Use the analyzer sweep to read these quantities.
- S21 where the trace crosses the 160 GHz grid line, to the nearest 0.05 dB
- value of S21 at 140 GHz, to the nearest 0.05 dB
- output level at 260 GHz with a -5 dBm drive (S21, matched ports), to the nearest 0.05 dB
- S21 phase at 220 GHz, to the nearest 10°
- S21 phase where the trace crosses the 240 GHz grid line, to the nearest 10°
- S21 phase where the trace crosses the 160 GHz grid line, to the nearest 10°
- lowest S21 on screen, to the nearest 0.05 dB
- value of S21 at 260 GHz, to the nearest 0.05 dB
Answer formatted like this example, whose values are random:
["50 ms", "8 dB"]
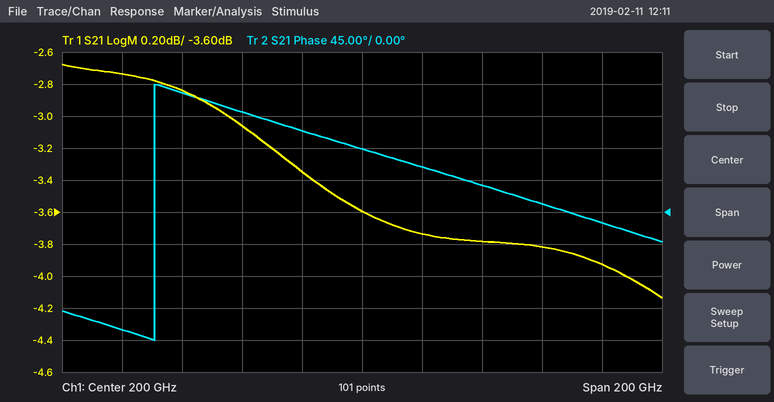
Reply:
["-3.05 dB", "-2.85 dB", "-8.80 dBm", "60°", "40°", "140°", "-4.15 dB", "-3.80 dB"]
